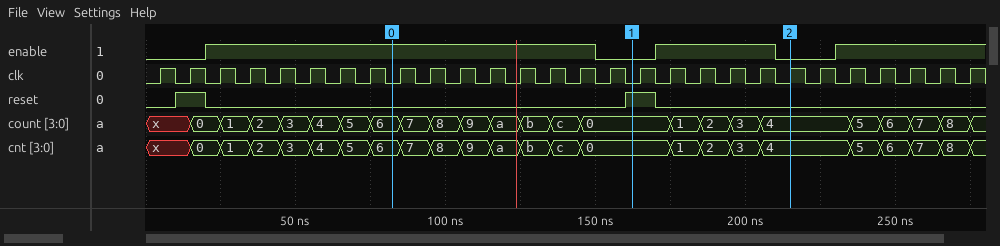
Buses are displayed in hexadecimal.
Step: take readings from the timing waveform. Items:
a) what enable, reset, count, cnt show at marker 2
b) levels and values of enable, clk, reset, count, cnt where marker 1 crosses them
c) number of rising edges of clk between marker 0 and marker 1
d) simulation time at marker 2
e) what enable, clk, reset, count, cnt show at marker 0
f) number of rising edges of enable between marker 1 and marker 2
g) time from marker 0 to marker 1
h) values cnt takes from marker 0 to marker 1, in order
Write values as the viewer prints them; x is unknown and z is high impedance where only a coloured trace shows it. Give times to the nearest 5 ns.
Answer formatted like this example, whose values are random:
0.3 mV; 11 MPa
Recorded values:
enable=0, reset=0, count=4, cnt=4; enable=0, clk=0, reset=1, count=0, cnt=0; 8; 215 ns; enable=1, clk=0, reset=0, count=6, cnt=6; 1; 80 ns; 6, 7, 8, 9, a, b, c, 0
